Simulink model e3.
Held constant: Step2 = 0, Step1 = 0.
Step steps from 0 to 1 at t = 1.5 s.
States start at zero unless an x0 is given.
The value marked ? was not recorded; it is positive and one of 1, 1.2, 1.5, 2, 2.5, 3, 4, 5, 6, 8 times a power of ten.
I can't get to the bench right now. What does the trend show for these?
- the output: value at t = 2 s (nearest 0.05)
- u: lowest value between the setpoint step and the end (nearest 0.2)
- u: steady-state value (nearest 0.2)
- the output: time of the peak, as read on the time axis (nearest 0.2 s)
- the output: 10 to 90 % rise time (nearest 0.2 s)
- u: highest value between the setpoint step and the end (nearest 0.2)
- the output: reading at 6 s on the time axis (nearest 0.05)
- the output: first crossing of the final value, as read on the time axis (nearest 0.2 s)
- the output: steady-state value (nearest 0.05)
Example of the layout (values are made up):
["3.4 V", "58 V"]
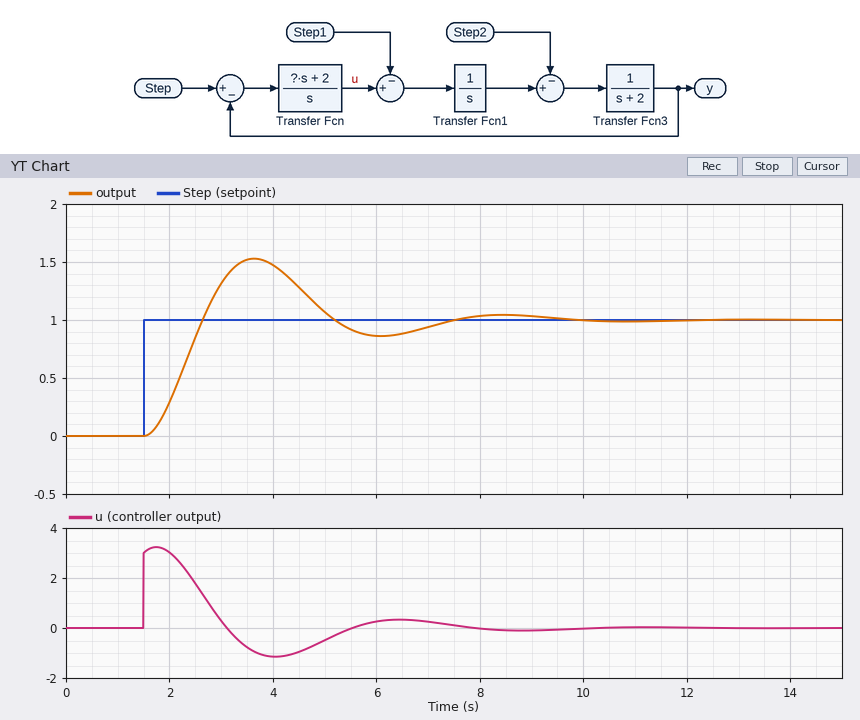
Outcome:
["0.30", "-1.2", "0.0", "3.6 s", "0.8 s", "3.2", "0.85", "2.6 s", "1.00"]
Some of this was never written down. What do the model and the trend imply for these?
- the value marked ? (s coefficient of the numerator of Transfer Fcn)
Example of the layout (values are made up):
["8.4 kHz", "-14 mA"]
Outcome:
["3"]
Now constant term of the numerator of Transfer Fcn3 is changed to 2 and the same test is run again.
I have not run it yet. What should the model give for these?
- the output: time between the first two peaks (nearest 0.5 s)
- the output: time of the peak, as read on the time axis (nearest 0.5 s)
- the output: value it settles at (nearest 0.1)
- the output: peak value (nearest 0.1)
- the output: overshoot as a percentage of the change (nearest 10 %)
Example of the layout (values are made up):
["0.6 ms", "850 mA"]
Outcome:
["3.0 s", "3.0 s", "1.0", "1.6", "60 %"]
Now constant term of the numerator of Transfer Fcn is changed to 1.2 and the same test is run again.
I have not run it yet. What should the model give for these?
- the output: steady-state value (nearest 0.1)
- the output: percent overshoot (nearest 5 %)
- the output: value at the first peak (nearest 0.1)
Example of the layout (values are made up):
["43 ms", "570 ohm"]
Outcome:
["1.0", "40 %", "1.4"]
